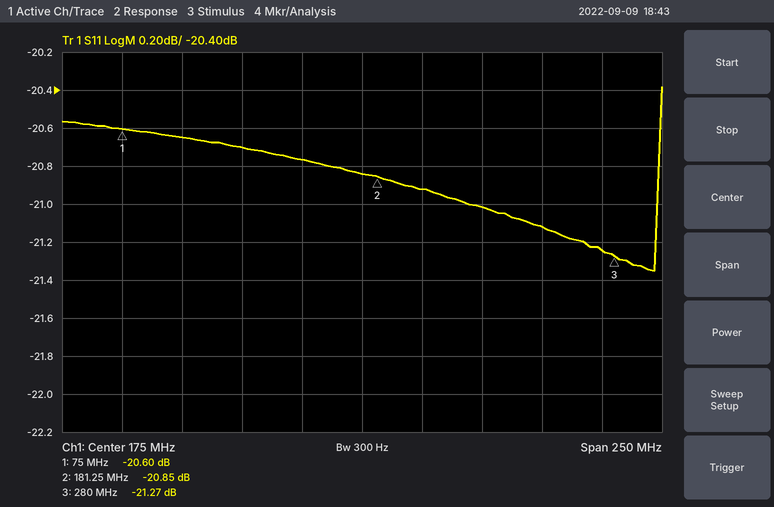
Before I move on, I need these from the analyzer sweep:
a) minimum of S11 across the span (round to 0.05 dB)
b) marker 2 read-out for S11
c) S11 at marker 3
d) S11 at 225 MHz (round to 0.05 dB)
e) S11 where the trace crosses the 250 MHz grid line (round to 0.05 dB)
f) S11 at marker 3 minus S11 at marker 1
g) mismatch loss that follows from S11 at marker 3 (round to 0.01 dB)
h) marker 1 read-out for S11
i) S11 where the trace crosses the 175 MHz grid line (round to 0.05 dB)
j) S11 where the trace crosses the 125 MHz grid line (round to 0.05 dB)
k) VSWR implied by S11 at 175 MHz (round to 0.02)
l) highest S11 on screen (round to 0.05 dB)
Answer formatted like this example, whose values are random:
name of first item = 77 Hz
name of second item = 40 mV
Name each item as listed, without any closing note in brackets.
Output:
minimum of S11 across the span = -21.35 dB
marker 2 read-out for S11 = -20.85 dB
S11 at marker 3 = -21.27 dB
S11 at 225 MHz = -21.00 dB
S11 where the trace crosses the 250 MHz grid line = -21.10 dB
S11 at marker 3 minus S11 at marker 1 = -0.67 dB
mismatch loss that follows from S11 at marker 3 = 0.03 dB
marker 1 read-out for S11 = -20.60 dB
S11 where the trace crosses the 175 MHz grid line = -20.85 dB
S11 where the trace crosses the 125 MHz grid line = -20.70 dB
VSWR implied by S11 at 175 MHz = 1.20
highest S11 on screen = -20.40 dB
